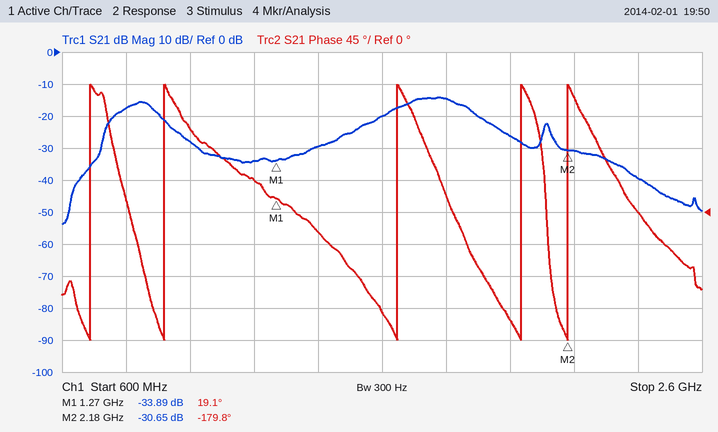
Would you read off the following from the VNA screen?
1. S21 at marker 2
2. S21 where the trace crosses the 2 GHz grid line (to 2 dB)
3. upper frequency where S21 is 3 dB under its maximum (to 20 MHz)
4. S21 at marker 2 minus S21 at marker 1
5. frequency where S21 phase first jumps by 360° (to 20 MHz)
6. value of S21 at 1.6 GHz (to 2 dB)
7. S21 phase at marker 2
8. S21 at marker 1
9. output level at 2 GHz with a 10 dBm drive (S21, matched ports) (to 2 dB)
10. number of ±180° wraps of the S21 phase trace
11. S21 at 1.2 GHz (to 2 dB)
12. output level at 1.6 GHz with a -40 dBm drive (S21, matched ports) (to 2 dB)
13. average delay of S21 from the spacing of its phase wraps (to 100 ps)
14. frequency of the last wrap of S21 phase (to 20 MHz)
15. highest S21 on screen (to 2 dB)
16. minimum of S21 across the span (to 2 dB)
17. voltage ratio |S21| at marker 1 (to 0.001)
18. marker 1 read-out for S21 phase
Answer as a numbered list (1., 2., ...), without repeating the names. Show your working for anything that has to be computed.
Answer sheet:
1. -30.65 dB
2. -26 dB
3. 1.86 GHz
4. -30.65 − (-33.89) = 3.24 dB
5. 680 MHz
6. -20 dB
7. -179.8°
8. -33.89 dB
9. 10 dBm + (-26 dB) = -16 dBm
10. 5
11. -34 dB
12. -40 dBm + (-20 dB) = -60 dBm
13. 4 cycles / (2.18 GHz − 680 MHz) ≈ 2.7 ns
14. 2.18 GHz
15. -14 dB
16. -54 dB
17. 10^(-33.89/20) ≈ 0.020
18. 19.1°
